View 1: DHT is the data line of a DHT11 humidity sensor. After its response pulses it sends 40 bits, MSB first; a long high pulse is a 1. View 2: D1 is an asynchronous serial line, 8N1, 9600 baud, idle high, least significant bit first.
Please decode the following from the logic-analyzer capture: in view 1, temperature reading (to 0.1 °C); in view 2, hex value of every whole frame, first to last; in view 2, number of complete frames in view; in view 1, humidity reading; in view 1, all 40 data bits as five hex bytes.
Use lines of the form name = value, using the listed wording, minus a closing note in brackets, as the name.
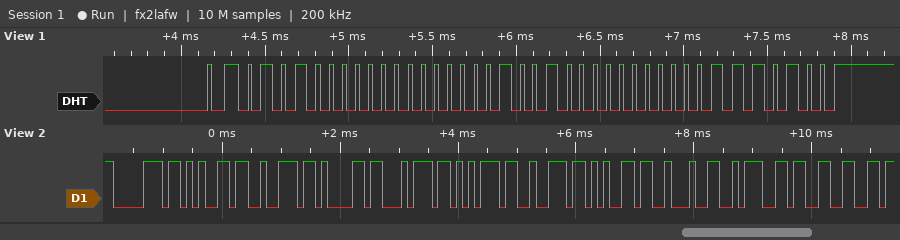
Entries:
in view 1, temperature reading = 36.0 °C
in view 2, hex value of every whole frame, first to last = 70 65 72 61 74 75 72 65 22 3A 33
in view 2, number of complete frames in view = 11
in view 1, humidity reading = 80 %
in view 1, all 40 data bits as five hex bytes = 50 00 24 00 74
